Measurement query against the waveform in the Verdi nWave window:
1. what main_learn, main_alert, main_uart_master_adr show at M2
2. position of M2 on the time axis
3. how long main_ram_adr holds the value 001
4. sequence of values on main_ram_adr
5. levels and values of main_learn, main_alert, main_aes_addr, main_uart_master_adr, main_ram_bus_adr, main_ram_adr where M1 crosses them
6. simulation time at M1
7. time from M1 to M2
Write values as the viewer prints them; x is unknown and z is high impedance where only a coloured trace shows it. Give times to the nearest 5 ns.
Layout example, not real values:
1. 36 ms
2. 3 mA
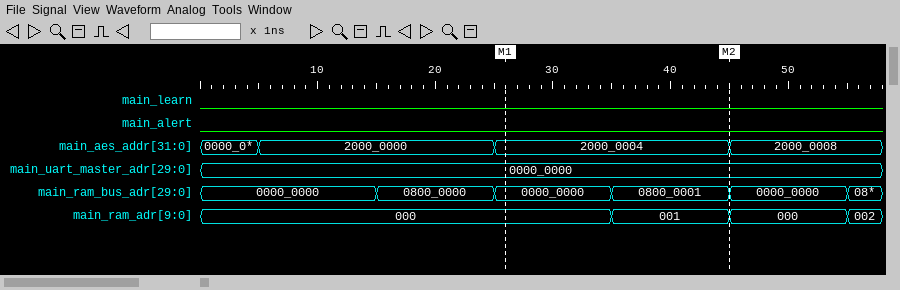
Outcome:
1. main_learn=0, main_alert=0, main_uart_master_adr=0000_0000
2. 45 ns
3. 10 ns
4. 000, 001, 000, 002
5. main_learn=0, main_alert=0, main_aes_addr=2000_0004, main_uart_master_adr=0000_0000, main_ram_bus_adr=0000_0000, main_ram_adr=000
6. 25 ns
7. 20 ns
